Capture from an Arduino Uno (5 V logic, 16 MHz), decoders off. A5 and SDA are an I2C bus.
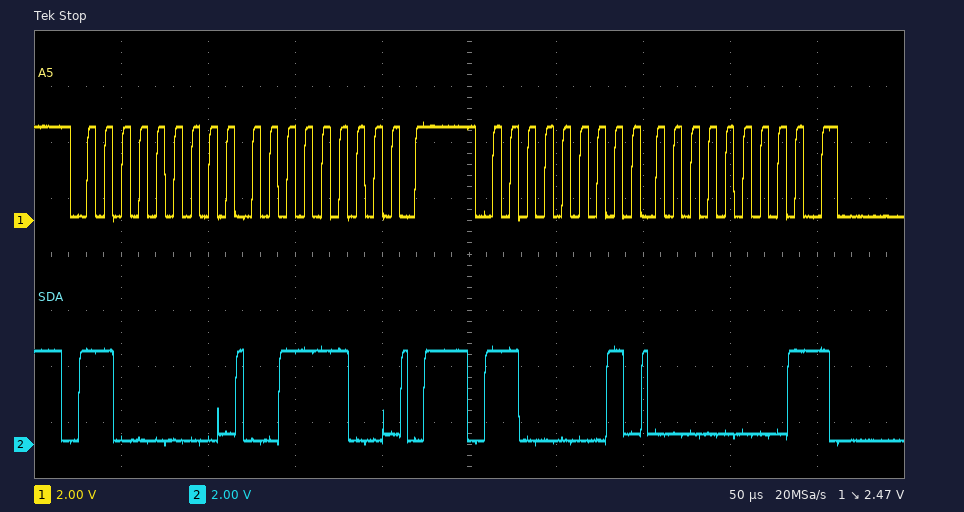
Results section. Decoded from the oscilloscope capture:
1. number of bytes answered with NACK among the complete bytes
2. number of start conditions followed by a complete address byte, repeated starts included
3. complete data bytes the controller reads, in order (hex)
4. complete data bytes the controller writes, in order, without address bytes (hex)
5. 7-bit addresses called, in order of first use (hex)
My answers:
1
2
00
3C
0x60
